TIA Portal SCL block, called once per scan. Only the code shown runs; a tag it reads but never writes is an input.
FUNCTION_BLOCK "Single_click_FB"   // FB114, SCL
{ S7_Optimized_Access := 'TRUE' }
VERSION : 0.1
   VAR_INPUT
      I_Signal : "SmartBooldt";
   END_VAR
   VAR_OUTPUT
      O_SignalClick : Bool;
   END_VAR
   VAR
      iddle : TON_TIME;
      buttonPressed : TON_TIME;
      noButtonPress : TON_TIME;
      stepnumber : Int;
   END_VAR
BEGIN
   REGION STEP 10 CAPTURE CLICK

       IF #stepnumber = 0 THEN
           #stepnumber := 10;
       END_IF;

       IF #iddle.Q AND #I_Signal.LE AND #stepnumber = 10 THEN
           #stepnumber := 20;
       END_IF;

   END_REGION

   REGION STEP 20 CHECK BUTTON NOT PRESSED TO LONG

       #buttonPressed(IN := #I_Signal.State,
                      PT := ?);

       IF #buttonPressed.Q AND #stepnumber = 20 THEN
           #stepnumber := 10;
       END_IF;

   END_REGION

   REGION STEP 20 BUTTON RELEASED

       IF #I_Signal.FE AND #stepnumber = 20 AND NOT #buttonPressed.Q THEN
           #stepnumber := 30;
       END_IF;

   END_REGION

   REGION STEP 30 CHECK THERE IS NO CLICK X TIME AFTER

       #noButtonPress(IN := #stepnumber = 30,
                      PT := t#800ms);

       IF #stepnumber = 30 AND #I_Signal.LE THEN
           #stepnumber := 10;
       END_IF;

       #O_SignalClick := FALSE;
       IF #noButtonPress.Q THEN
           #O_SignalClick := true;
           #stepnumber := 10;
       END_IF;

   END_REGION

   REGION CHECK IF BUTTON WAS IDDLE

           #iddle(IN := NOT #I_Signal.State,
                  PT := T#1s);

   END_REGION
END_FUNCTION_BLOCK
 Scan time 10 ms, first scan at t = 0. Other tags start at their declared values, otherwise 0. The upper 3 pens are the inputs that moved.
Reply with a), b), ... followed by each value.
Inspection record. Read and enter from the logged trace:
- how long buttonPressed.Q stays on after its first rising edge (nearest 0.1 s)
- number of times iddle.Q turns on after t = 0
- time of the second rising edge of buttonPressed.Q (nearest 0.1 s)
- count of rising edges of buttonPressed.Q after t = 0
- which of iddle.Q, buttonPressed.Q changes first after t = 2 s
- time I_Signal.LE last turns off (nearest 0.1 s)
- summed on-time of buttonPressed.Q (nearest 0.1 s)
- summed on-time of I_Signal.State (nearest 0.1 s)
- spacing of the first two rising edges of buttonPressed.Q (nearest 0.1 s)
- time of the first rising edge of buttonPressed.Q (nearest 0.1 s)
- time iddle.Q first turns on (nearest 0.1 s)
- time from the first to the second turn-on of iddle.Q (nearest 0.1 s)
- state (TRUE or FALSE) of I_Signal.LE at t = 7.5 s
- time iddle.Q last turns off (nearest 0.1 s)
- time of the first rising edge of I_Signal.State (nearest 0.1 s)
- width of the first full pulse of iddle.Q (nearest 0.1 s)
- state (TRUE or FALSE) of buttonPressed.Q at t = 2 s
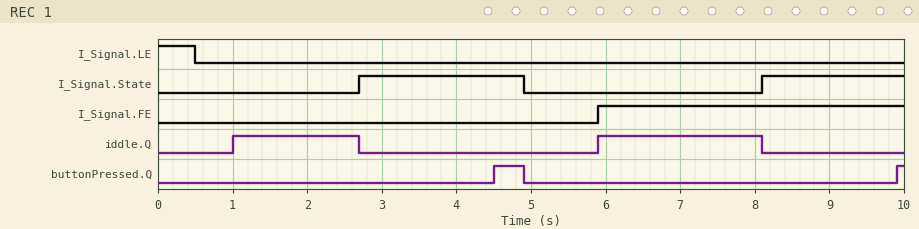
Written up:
a) 0.4 s
b) 2
c) 9.9 s
d) 2
e) iddle.Q
f) 0.5 s
g) 0.5 s
h) 4.1 s
i) 5.4 s
j) 4.5 s
k) 1.0 s
l) 4.9 s
m) FALSE
n) 8.1 s
o) 2.7 s
p) 1.7 s
q) FALSE
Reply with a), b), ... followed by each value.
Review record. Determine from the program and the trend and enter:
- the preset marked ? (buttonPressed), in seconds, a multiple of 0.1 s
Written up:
a) 1.8 s
